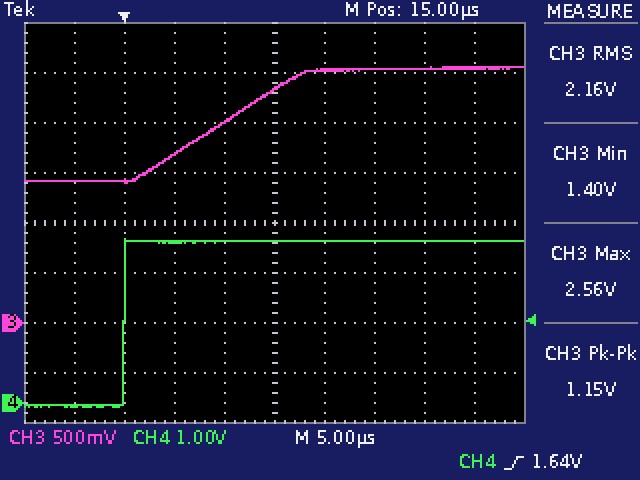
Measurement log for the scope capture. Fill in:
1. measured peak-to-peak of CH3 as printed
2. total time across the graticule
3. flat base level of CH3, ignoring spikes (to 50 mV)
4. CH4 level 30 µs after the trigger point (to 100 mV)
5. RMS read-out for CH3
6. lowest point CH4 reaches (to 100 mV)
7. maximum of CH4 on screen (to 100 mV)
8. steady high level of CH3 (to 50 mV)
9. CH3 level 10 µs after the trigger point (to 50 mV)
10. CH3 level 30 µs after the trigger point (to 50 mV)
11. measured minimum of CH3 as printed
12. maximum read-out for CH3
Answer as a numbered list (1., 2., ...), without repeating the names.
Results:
1. 1.15 V
2. 50 µs
3. 1.40 V
4. 3.2 V
5. 2.16 V
6. -100 mV
7. 3.3 V
8. 2.55 V
9. 2.00 V
10. 2.55 V
11. 1.40 V
12. 2.56 V
